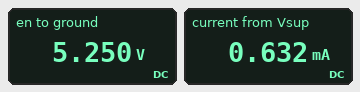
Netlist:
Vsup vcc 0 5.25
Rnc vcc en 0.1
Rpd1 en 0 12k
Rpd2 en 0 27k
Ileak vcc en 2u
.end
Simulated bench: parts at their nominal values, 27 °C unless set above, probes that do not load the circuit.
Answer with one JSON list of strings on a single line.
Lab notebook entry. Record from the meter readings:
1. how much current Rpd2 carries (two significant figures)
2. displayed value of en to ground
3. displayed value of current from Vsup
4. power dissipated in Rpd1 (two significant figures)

["190 µA", "5.250 V", "0.632 mA", "2.3 mW"]
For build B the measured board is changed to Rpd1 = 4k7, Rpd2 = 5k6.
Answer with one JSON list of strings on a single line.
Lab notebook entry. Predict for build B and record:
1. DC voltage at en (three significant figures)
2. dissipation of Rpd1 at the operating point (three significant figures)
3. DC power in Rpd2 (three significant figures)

["5.25 V", "5.86 mW", "4.92 mW"]
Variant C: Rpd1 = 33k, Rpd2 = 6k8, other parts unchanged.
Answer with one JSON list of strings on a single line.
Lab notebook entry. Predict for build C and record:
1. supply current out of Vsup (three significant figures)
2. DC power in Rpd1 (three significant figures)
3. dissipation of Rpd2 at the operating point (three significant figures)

["931 µA", "835 µW", "4.05 mW"]
